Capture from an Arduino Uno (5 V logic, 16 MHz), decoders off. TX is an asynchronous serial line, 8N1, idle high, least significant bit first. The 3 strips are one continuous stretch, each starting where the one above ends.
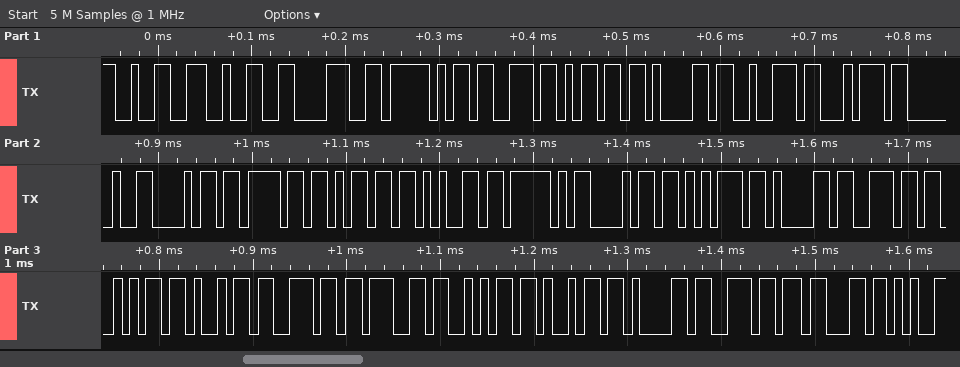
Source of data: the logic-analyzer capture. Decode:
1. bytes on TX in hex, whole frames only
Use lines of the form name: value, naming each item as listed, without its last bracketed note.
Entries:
bytes on TX in hex, whole frames only: 32 32 38 5F 73 6D 61 72 74 20 68 6F 6D 65 5F 68 75 61 6E 6A 69 6E 67 6A 69 61 6E 63
